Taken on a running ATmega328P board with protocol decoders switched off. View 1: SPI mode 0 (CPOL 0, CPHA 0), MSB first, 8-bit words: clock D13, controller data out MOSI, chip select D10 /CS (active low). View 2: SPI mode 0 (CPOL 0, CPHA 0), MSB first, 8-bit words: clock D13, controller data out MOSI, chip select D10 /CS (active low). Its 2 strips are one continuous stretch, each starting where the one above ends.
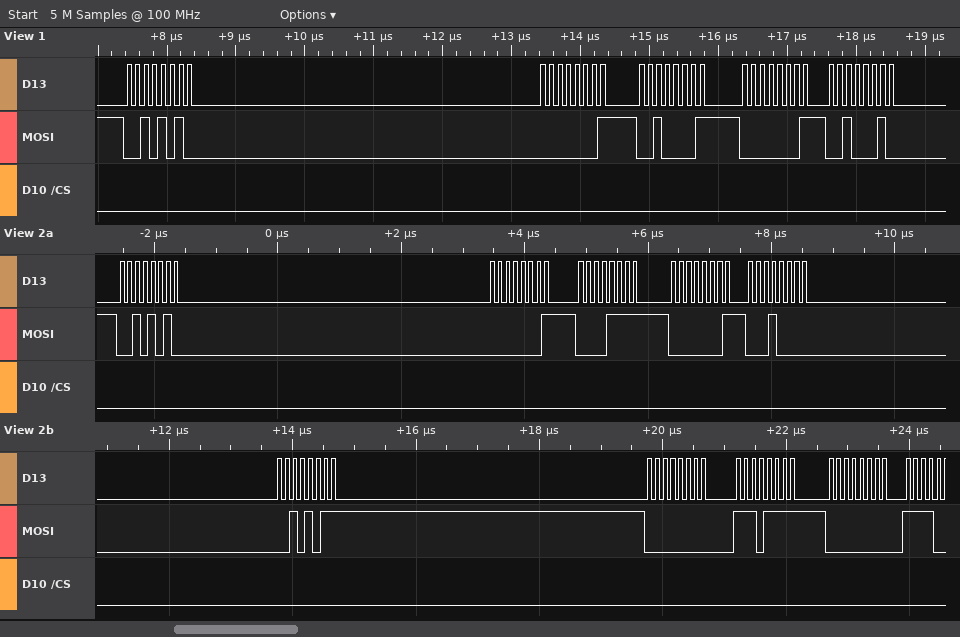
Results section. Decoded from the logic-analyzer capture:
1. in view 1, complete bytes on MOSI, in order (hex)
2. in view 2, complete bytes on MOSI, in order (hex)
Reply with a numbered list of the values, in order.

1. 2A 01 21 01 22
2. 0x2A 0x01 0x0F 0x01 0x10 0x2B 0x00 0xEF 0x00
